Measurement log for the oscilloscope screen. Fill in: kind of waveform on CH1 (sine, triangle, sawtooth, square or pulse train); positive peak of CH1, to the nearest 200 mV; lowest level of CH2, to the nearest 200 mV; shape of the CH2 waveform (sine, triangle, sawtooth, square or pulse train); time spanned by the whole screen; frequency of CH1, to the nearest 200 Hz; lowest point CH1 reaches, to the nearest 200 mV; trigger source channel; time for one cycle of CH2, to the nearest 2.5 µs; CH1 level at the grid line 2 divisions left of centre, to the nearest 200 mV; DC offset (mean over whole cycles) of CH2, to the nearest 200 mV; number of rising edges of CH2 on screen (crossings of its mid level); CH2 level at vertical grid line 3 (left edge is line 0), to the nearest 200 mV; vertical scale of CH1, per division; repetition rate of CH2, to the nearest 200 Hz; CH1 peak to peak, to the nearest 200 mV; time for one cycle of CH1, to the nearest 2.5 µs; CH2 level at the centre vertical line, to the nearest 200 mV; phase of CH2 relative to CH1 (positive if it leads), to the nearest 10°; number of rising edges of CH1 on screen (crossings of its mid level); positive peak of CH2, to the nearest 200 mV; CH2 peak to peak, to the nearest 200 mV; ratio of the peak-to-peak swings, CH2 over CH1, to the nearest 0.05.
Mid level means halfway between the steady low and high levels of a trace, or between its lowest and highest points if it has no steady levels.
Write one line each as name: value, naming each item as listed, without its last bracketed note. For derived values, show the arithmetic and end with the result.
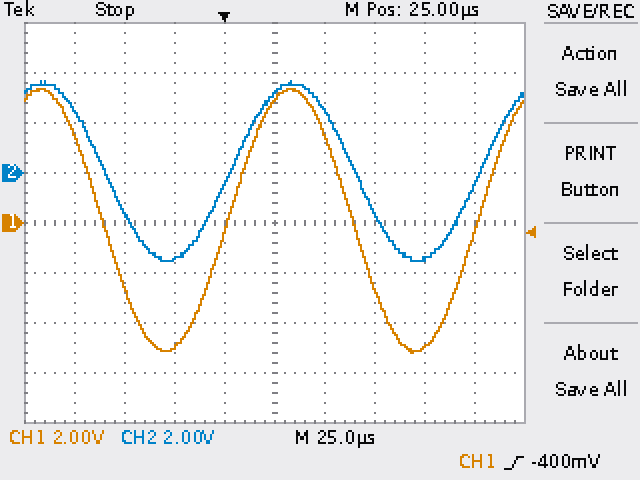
kind of waveform on CH1: sine
positive peak of CH1, to the nearest 200 mV: 5.4 V
lowest level of CH2, to the nearest 200 mV: -3.6 V
shape of the CH2 waveform: sine
time spanned by the whole screen: 250 µs
frequency of CH1, to the nearest 200 Hz: 1 / 125.0 µs ≈ 8.0 kHz
lowest point CH1 reaches, to the nearest 200 mV: -5.2 V
trigger source channel: CH1
time for one cycle of CH2, to the nearest 2.5 µs: 125.0 µs
CH1 level at the grid line 2 divisions left of centre, to the nearest 200 mV: -5.0 V
DC offset (mean over whole cycles) of CH2, to the nearest 200 mV: (3.6 V + (-3.6 V)) / 2 ≈ 0.0 V
number of rising edges of CH2 on screen: 2
CH2 level at vertical grid line 3 (left edge is line 0), to the nearest 200 mV: -3.4 V
vertical scale of CH1, per division: 2 V
repetition rate of CH2, to the nearest 200 Hz: 1 / 125.0 µs ≈ 8.0 kHz
CH1 peak to peak, to the nearest 200 mV: 5.4 V − (-5.2 V) = 10.6 V
time for one cycle of CH1, to the nearest 2.5 µs: 125.0 µs
CH2 level at the centre vertical line, to the nearest 200 mV: 3.2 V
phase of CH2 relative to CH1 (positive if it leads), to the nearest 10°: 0°
number of rising edges of CH1 on screen: 2
positive peak of CH2, to the nearest 200 mV: 3.6 V
CH2 peak to peak, to the nearest 200 mV: 3.6 V − (-3.6 V) = 7.2 V
ratio of the peak-to-peak swings, CH2 over CH1, to the nearest 0.05: 7.2 V / 10.6 V ≈ 0.679, so 0.70 to the nearest 0.05
